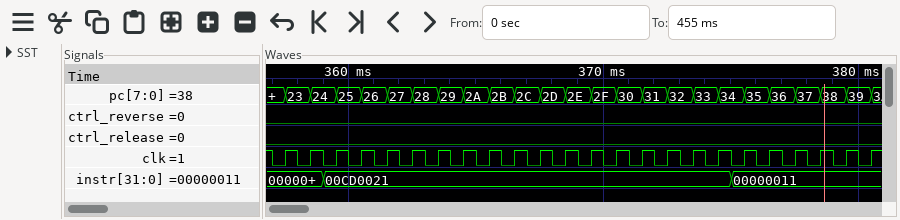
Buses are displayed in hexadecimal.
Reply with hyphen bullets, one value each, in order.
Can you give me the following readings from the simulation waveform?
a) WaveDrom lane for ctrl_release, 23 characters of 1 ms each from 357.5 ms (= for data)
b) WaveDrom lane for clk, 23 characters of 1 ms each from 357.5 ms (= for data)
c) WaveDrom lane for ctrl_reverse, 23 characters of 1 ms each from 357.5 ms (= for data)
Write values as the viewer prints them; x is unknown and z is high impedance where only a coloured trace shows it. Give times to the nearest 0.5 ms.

- {name: 'ctrl_release', wave: '0......................'}
- {name: 'clk', wave: 'p......................'}
- {name: 'ctrl_reverse', wave: '0......................'}
